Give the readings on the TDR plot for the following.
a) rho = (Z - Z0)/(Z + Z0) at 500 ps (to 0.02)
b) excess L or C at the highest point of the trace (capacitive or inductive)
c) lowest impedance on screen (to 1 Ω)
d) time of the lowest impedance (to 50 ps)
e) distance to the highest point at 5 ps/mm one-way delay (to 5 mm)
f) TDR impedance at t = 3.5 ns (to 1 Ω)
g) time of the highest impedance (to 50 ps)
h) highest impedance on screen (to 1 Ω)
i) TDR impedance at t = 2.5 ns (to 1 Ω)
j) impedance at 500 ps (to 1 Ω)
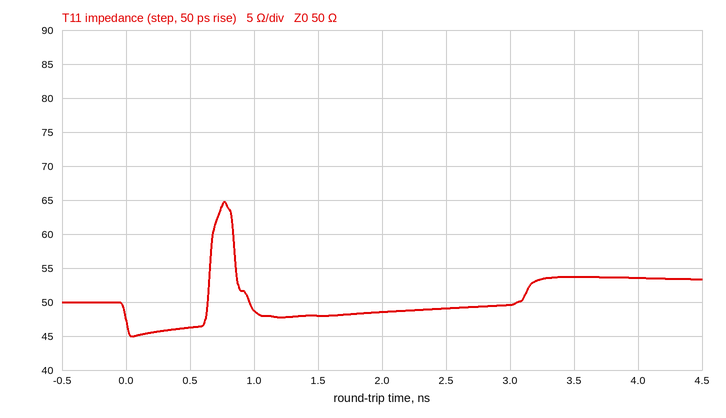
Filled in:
-0.04
inductive
45 Ω
50 ps
75 mm
54 Ω
750 ps
65 Ω
49 Ω
46 Ω
